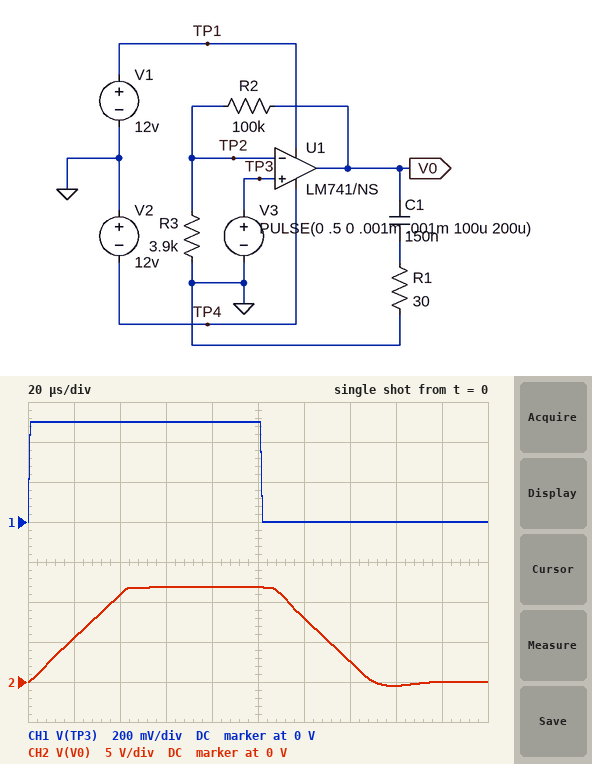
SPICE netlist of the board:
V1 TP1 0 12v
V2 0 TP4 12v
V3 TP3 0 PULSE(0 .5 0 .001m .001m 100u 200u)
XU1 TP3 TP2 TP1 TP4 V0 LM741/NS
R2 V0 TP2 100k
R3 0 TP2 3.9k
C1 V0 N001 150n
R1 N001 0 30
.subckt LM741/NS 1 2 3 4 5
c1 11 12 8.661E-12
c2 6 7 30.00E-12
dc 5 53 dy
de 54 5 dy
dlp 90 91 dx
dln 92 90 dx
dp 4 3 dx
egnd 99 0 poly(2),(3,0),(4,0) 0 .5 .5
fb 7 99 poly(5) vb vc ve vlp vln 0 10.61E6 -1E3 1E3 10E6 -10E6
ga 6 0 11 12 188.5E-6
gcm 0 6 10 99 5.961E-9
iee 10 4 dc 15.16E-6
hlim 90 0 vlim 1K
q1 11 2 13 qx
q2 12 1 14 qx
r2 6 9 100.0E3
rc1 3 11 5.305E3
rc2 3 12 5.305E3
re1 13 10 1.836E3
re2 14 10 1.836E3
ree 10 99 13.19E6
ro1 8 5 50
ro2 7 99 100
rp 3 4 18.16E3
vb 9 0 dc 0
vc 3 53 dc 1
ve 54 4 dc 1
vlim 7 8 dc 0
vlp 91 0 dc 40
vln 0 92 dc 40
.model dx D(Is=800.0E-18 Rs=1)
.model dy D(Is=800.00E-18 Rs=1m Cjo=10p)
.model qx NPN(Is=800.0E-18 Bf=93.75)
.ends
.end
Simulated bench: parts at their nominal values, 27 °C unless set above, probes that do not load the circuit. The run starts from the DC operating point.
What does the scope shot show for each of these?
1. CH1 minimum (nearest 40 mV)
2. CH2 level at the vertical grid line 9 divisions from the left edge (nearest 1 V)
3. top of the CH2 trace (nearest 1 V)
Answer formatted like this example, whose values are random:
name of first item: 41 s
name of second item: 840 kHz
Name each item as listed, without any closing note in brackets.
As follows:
CH1 minimum: 0 V
CH2 level at the vertical grid line 9 divisions from the left edge: 0 V
top of the CH2 trace: 12 V
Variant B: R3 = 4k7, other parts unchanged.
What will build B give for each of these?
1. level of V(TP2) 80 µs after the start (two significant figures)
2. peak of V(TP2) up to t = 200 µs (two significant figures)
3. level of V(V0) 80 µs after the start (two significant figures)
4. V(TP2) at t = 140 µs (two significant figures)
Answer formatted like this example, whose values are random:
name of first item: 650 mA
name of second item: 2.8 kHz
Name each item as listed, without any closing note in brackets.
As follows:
level of V(TP2) 80 µs after the start: 500 mV
peak of V(TP2) up to t = 200 µs: 520 mV
level of V(V0) 80 µs after the start: 11 V
V(TP2) at t = 140 µs: 23 mV
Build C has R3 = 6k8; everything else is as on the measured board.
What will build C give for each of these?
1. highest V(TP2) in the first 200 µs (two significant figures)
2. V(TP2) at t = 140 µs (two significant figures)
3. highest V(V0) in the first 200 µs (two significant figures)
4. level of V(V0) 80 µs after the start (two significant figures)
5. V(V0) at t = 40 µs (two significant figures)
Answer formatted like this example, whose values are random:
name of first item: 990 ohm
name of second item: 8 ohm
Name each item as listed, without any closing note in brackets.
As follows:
highest V(TP2) in the first 200 µs: 530 mV
V(TP2) at t = 140 µs: -23 mV
highest V(V0) in the first 200 µs: 8.3 V
level of V(V0) 80 µs after the start: 7.9 V
V(V0) at t = 40 µs: 8.2 V
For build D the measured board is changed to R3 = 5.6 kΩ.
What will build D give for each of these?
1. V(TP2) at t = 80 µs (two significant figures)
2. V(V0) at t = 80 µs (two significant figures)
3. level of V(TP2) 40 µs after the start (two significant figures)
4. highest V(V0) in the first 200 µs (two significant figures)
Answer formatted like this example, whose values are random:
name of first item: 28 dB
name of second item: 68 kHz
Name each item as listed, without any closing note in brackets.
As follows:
V(TP2) at t = 80 µs: 500 mV
V(V0) at t = 80 µs: 9.4 V
level of V(TP2) 40 µs after the start: 520 mV
highest V(V0) in the first 200 µs: 9.9 V
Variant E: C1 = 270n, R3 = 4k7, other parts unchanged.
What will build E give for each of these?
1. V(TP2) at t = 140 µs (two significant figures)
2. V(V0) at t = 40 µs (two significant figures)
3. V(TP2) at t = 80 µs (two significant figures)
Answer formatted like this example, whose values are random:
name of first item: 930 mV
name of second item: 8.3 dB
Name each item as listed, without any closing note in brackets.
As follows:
V(TP2) at t = 140 µs: 210 mV
V(V0) at t = 40 µs: 6.7 V
V(TP2) at t = 80 µs: 520 mV
